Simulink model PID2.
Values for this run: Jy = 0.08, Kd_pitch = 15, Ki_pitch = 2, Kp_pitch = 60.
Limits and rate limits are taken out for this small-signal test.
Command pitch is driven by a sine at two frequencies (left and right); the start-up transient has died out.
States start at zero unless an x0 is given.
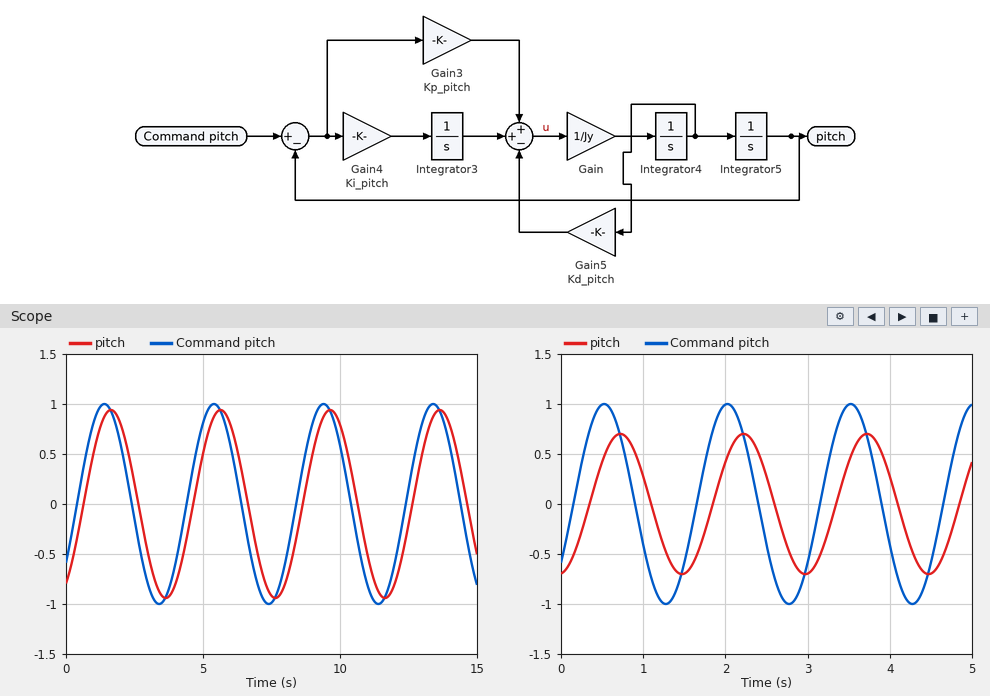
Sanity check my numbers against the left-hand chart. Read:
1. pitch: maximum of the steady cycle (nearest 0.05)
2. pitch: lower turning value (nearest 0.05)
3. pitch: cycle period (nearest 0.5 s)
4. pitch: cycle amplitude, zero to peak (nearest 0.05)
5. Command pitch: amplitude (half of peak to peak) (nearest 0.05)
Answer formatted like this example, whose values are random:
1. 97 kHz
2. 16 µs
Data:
1. 0.95
2. -0.95
3. 4.0 s
4. 0.95
5. 1.00
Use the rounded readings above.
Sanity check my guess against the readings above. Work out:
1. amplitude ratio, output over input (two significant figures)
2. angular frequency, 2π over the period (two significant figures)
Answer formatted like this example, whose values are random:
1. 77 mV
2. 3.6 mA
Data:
1. 0.95
2. 1.6 rad/s
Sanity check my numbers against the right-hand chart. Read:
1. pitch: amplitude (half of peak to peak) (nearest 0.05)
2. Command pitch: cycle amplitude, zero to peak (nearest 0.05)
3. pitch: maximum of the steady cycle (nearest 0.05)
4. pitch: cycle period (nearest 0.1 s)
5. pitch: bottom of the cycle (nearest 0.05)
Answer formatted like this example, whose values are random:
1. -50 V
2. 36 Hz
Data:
1. 0.70
2. 1.00
3. 0.70
4. 1.5 s
5. -0.70
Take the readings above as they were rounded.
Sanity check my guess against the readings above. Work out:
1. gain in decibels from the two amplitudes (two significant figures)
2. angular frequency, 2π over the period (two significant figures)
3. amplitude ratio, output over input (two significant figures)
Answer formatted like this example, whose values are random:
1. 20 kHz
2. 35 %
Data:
1. -3.1 dB
2. 4.2 rad/s
3. 0.70
